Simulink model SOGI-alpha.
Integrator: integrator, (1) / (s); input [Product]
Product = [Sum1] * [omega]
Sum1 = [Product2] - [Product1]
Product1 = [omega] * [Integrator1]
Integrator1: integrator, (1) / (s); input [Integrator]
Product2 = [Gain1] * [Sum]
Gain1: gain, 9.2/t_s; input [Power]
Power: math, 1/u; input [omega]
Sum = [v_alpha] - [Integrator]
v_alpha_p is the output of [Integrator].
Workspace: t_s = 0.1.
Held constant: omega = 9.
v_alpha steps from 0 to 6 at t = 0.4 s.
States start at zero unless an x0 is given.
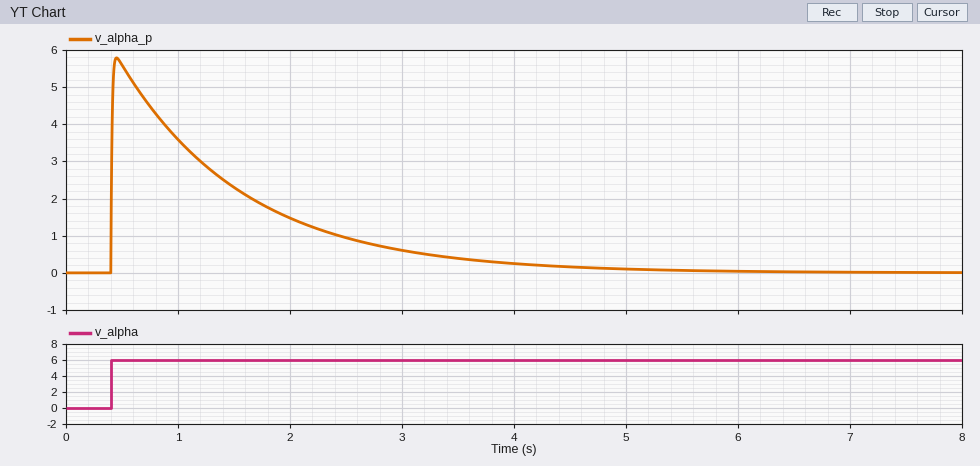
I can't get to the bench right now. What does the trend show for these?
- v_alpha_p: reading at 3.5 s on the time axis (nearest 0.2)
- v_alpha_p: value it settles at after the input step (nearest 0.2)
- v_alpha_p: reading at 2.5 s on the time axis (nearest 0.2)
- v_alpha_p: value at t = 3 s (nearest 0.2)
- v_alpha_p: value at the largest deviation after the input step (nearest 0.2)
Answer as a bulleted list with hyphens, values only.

- 0.4
- 0.0
- 1.0
- 0.6
- 5.8
